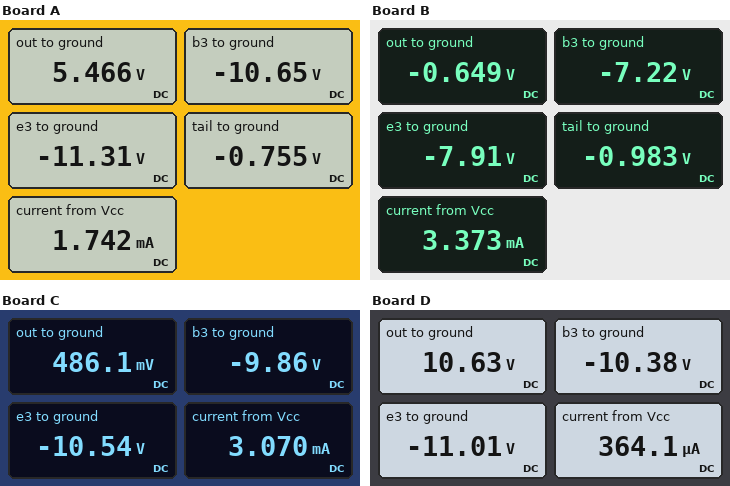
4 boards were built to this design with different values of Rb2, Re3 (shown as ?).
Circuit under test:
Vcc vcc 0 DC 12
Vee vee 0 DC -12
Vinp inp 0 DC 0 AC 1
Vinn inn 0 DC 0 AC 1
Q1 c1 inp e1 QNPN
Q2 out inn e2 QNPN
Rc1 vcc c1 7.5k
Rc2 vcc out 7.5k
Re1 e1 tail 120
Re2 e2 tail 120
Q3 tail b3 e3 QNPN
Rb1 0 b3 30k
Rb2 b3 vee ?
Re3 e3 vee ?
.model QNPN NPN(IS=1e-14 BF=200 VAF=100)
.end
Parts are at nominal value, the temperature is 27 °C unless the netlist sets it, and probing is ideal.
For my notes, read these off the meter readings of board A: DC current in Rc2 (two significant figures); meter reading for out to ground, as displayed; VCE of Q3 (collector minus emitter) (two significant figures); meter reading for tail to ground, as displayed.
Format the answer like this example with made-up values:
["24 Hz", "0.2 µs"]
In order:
["870 µA", "5.466 V", "11 V", "-0.755 V"]
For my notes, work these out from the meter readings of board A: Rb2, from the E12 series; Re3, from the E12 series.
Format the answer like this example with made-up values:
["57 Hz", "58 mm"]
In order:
["3.9 kΩ", "390 Ω"]
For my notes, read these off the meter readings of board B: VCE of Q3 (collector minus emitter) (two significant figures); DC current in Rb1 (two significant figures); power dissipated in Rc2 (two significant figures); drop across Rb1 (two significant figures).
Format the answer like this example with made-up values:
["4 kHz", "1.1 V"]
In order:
["6.9 V", "240 µA", "21 mW", "7.2 V"]
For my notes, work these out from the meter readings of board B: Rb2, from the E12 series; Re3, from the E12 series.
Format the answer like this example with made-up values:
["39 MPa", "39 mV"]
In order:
["22 kΩ", "820 Ω"]
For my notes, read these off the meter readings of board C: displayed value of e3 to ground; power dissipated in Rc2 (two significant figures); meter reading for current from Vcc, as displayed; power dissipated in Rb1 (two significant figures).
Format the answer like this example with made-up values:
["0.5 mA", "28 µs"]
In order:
["-10.54 V", "18 mW", "3.070 mA", "3.2 mW"]
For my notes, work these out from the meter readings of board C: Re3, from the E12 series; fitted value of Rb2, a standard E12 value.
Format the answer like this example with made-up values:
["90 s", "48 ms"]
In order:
["470 Ω", "6.8 kΩ"]
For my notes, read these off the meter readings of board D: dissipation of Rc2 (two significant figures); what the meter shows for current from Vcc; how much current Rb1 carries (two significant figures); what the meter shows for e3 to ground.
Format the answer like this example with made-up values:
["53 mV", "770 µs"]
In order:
["250 µW", "364.1 µA", "350 µA", "-11.01 V"]
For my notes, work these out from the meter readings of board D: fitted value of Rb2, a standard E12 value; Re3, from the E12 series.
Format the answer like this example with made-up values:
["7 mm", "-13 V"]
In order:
["4.7 kΩ", "2.7 kΩ"]
